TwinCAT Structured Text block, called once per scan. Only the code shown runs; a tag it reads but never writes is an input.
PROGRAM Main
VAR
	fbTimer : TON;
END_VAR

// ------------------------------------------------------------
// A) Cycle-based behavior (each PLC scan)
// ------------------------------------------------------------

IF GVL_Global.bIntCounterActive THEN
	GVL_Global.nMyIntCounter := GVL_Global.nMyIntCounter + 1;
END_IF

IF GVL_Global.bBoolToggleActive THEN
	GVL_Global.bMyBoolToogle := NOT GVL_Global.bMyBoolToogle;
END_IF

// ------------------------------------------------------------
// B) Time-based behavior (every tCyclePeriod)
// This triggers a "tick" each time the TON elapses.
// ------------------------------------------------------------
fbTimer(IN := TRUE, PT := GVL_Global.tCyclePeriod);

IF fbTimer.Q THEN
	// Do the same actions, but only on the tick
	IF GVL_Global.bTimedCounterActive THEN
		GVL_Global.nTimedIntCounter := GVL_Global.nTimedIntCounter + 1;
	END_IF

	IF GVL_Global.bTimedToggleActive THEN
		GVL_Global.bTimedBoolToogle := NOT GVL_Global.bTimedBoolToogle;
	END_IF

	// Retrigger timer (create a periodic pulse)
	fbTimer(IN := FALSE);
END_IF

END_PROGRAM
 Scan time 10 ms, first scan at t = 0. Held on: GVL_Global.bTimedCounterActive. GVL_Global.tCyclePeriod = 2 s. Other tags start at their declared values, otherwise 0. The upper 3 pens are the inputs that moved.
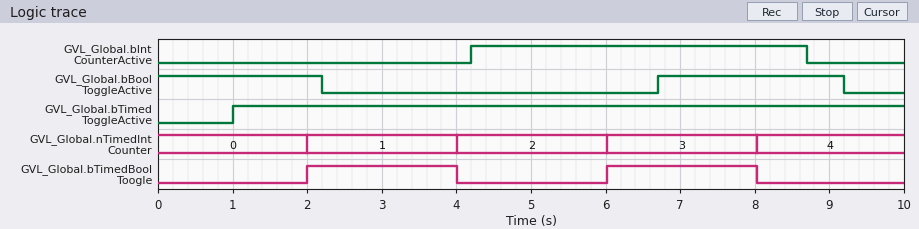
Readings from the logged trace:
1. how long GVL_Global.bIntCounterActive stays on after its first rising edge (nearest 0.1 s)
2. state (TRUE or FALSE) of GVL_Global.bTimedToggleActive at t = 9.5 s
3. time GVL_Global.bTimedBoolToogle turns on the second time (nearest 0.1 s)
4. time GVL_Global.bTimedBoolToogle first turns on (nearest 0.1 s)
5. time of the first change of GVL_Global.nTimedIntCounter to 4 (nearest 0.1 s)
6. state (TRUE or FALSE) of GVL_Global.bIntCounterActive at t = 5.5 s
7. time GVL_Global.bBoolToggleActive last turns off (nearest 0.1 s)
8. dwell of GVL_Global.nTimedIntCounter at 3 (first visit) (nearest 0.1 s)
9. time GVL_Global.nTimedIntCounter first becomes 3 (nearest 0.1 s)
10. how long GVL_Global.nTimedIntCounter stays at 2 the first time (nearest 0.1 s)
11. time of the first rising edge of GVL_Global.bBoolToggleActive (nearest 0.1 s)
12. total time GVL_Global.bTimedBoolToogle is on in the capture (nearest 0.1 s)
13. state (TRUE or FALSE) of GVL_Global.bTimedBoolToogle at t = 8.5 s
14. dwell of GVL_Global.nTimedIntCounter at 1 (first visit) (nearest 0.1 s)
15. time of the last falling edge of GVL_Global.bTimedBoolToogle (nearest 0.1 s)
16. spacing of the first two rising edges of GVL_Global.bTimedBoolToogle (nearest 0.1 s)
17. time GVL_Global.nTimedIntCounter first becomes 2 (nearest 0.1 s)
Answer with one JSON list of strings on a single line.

["4.5 s", "TRUE", "6.0 s", "2.0 s", "8.0 s", "TRUE", "9.2 s", "2.0 s", "6.0 s", "2.0 s", "6.7 s", "4.0 s", "FALSE", "2.0 s", "8.0 s", "4.0 s", "4.0 s"]
